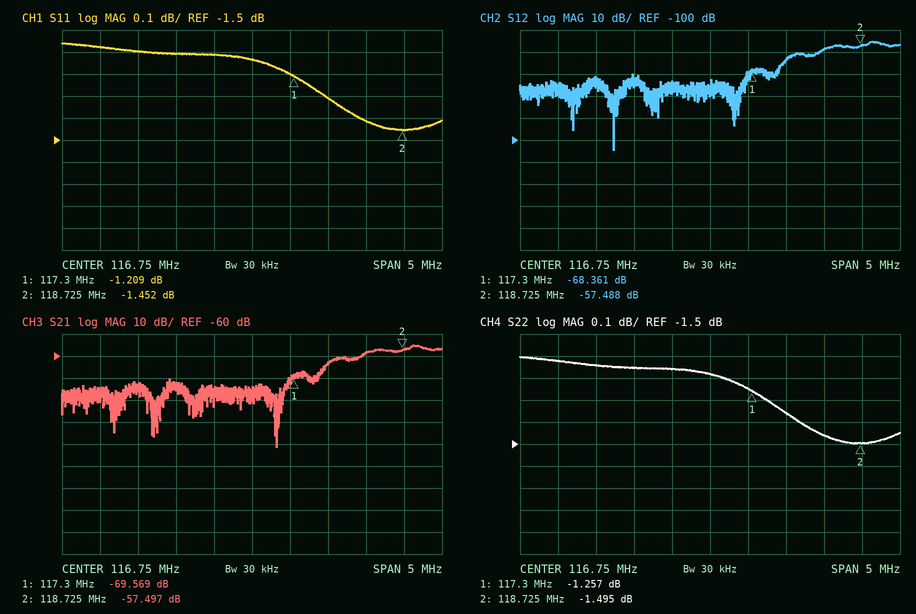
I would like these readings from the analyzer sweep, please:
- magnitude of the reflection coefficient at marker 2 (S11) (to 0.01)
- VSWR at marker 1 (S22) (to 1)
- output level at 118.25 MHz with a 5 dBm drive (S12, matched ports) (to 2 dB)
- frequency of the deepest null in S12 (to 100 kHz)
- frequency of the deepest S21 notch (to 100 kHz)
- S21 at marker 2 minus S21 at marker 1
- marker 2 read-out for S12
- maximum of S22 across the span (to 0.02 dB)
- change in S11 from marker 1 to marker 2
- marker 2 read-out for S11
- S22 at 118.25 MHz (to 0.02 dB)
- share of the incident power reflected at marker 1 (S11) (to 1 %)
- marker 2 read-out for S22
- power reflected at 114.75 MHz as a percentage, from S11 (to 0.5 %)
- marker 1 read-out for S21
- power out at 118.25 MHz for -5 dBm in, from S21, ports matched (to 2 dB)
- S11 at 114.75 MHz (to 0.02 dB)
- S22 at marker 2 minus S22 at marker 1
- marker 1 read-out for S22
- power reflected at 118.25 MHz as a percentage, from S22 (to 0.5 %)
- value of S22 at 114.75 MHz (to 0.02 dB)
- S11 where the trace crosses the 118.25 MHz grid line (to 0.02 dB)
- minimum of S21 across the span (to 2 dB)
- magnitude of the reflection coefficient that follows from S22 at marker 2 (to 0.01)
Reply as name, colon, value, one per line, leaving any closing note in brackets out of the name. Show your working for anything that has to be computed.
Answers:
magnitude of the reflection coefficient at marker 2 (S11): 10^(-1.452/20) ≈ 0.85
VSWR at marker 1 (S22): (1 + 0.8653)/(1 − 0.8653) ≈ 14
output level at 118.25 MHz with a 5 dBm drive (S12, matched ports): 5 dBm + (-58 dB) = -54 dBm
frequency of the deepest null in S12: 115.5 MHz
frequency of the deepest S21 notch: 117.1 MHz
S21 at marker 2 minus S21 at marker 1: -57.497 − (-69.569) = 12.072 dB
marker 2 read-out for S12: -57.488 dB
maximum of S22 across the span: -1.10 dB
change in S11 from marker 1 to marker 2: -1.452 − (-1.209) = -0.243 dB
marker 2 read-out for S11: -1.452 dB
S22 at 118.25 MHz: -1.46 dB
share of the incident power reflected at marker 1 (S11): 10^(-1.209/10) ≈ 76 %
marker 2 read-out for S22: -1.495 dB
power reflected at 114.75 MHz as a percentage, from S11: 10^(-1.08/10) ≈ 78.0 %
marker 1 read-out for S21: -69.569 dB
power out at 118.25 MHz for -5 dBm in, from S21, ports matched: -5 dBm + (-58 dB) = -64 dBm
S11 at 114.75 MHz: -1.08 dB
S22 at marker 2 minus S22 at marker 1: -1.495 − (-1.257) = -0.238 dB
marker 1 read-out for S22: -1.257 dB
power reflected at 118.25 MHz as a percentage, from S22: 10^(-1.46/10) ≈ 71.4 %, so 71.5 % to the nearest 0.5 %
value of S22 at 114.75 MHz: -1.12 dB
S11 where the trace crosses the 118.25 MHz grid line: -1.42 dB
minimum of S21 across the span: -102 dB
magnitude of the reflection coefficient that follows from S22 at marker 2: 10^(-1.495/20) ≈ 0.84
